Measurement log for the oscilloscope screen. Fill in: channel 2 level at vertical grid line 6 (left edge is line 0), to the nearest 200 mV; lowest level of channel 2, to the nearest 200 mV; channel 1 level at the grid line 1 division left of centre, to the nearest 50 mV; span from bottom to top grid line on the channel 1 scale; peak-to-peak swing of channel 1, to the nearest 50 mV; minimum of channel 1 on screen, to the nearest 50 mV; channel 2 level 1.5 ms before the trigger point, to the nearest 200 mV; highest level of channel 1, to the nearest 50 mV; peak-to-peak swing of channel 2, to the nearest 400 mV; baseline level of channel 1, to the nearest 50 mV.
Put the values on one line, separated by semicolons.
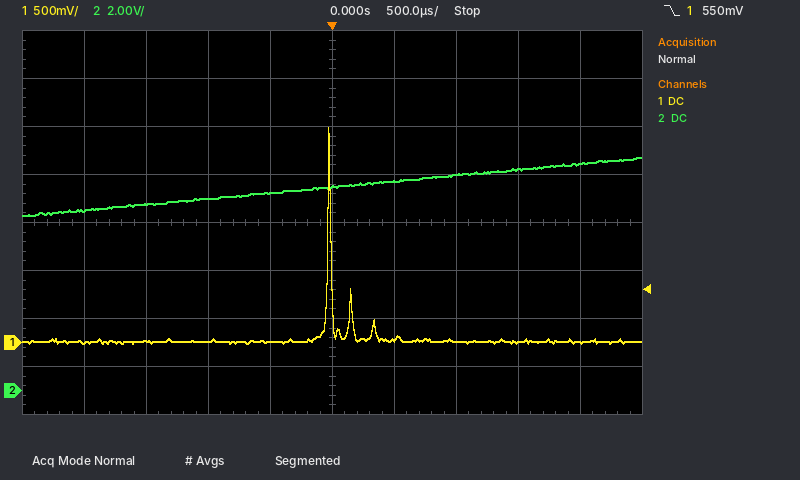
8.8 V; 7.2 V; 0 mV; 4 V; 2.25 V; 0 mV; 7.8 V; 2.25 V; 2.4 V; 0 mV
